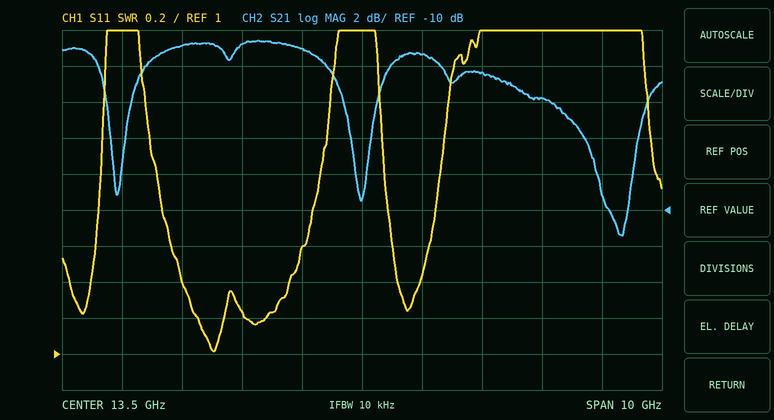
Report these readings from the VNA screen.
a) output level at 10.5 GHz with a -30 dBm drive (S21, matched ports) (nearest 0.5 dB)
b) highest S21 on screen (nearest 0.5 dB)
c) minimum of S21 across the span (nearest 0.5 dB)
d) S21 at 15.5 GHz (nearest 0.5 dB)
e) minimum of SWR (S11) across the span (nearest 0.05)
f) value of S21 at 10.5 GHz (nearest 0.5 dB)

-31.0 dBm
-0.5 dB
-11.5 dB
-2.5 dB
1.00
-1.0 dB
